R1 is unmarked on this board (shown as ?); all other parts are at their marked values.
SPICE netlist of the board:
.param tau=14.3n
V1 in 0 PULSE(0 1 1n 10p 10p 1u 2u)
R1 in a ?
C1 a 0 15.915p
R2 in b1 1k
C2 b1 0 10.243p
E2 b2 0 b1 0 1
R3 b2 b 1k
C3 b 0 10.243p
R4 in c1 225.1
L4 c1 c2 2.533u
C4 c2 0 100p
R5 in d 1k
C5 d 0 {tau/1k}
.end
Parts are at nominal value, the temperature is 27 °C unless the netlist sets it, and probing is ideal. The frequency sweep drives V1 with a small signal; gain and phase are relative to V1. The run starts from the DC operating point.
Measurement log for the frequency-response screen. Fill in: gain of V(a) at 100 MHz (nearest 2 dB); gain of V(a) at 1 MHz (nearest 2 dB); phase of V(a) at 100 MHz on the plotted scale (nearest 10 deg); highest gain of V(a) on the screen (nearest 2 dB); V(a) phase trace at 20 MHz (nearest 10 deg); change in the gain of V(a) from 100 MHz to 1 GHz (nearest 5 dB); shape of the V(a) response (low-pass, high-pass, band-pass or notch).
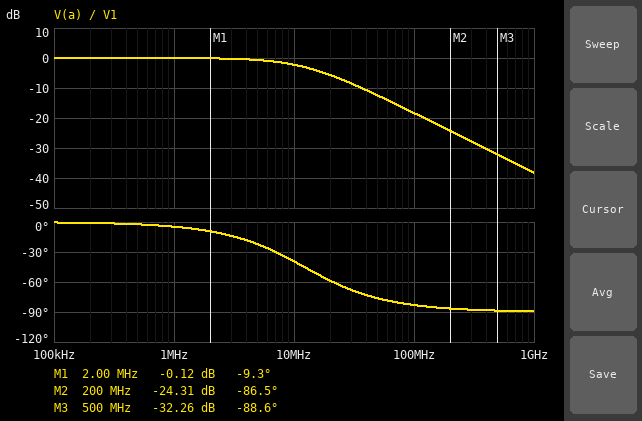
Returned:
-18 dB
0 dB
-80 deg
0 dB
-60 deg
-20 dB
low-pass
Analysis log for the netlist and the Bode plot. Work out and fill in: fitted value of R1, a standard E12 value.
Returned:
820 Ω
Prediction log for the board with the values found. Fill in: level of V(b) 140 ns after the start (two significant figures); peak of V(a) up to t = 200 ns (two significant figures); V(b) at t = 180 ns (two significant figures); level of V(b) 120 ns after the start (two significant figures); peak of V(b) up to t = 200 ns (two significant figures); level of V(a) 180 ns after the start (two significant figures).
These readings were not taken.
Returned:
1.0 V
1.0 V
1.0 V
1.0 V
1.0 V
1.0 V
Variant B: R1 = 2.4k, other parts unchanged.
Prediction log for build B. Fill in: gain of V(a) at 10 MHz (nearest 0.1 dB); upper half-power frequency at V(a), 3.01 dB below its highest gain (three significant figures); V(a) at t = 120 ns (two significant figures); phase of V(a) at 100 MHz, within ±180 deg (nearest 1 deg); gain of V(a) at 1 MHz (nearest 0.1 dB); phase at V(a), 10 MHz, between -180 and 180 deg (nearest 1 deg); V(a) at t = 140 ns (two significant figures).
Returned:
-8.3 dB
4.17 MHz
960 mV
-88 deg
-0.2 dB
-67 deg
970 mV
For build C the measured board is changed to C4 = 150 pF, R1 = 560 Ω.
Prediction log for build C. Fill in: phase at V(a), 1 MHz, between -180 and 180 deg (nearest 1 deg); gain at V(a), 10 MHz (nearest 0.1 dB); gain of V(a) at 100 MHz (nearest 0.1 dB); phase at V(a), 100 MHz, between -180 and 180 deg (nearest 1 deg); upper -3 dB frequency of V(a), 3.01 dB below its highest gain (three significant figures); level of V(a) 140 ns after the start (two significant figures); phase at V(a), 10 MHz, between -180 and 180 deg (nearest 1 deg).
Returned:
-3 deg
-1.2 dB
-15.1 dB
-80 deg
17.9 MHz
1.0 V
-29 deg
